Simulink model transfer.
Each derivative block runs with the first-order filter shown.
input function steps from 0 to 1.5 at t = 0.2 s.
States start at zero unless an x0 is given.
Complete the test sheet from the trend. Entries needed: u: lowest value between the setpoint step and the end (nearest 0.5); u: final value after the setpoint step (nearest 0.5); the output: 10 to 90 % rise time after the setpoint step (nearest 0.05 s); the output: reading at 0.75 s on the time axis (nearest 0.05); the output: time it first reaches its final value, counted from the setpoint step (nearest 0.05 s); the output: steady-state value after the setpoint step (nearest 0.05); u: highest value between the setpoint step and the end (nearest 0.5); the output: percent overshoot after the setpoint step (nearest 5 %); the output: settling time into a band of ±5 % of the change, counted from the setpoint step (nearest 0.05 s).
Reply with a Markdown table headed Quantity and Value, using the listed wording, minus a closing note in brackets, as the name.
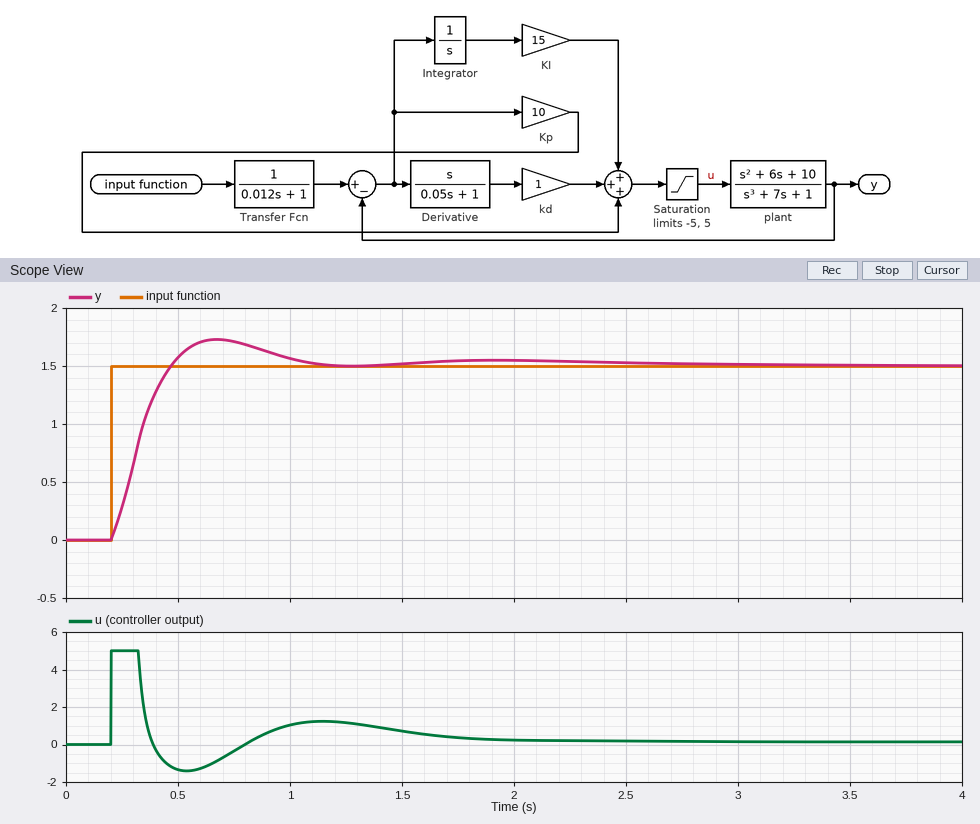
| Quantity | Value |
|---|---|
| u: lowest value between the setpoint step and the end | -1.5 |
| u: final value after the setpoint step | 0.0 |
| the output: 10 to 90 % rise time after the setpoint step | 0.20 s |
| the output: reading at 0.75 s on the time axis | 1.70 |
| the output: time it first reaches its final value, counted from the setpoint step | 0.25 s |
| the output: steady-state value after the setpoint step | 1.50 |
| u: highest value between the setpoint step and the end | 5.0 |
| the output: percent overshoot after the setpoint step | 15 % |
| the output: settling time into a band of ±5 % of the change, counted from the setpoint step | 0.80 s |
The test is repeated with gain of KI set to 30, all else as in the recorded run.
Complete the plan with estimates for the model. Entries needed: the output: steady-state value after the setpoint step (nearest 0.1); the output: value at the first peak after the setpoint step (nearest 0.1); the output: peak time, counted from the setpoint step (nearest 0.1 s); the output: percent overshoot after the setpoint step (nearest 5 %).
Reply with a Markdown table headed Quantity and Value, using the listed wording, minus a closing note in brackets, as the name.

| Quantity | Value |
|---|---|
| the output: steady-state value after the setpoint step | 1.5 |
| the output: value at the first peak after the setpoint step | 1.9 |
| the output: peak time, counted from the setpoint step | 0.4 s |
| the output: percent overshoot after the setpoint step | 25 % |
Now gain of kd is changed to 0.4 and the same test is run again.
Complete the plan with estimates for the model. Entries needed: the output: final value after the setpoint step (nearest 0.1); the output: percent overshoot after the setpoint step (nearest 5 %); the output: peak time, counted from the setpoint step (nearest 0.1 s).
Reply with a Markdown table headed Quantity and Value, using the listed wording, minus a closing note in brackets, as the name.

| Quantity | Value |
|---|---|
| the output: final value after the setpoint step | 1.5 |
| the output: percent overshoot after the setpoint step | 25 % |
| the output: peak time, counted from the setpoint step | 0.4 s |
